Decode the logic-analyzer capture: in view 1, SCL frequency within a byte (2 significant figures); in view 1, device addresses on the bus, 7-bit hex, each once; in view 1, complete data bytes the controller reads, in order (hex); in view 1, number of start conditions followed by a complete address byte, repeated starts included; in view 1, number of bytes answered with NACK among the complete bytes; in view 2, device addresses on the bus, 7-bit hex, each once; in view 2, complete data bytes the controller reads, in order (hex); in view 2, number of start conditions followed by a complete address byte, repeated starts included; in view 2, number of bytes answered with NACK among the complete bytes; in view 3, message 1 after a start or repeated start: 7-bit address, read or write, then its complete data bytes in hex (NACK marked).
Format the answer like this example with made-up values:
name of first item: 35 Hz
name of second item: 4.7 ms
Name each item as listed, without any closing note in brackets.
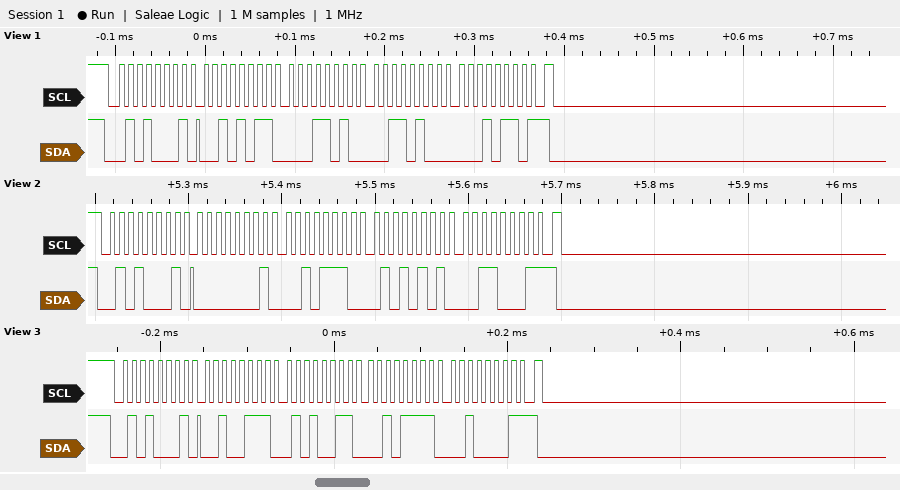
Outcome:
in view 1, SCL frequency within a byte: 100 kHz
in view 1, device addresses on the bus, 7-bit hex, each once: 0x28
in view 1, complete data bytes the controller reads, in order: 2B 1A 34 16
in view 1, number of start conditions followed by a complete address byte, repeated starts included: 1
in view 1, number of bytes answered with NACK among the complete bytes: 1
in view 2, device addresses on the bus, 7-bit hex, each once: 0x28
in view 2, complete data bytes the controller reads, in order: 01 2E 55 31
in view 2, number of start conditions followed by a complete address byte, repeated starts included: 1
in view 2, number of bytes answered with NACK among the complete bytes: 1
in view 3, message 1 after a start or repeated start: 7-bit address, read or write, then its complete data bytes in hex: 0x28 read: 27 53 2F 21 NACK
